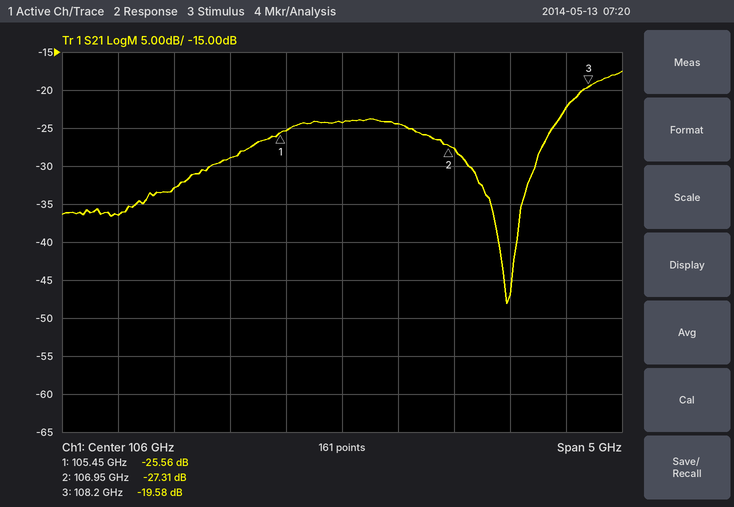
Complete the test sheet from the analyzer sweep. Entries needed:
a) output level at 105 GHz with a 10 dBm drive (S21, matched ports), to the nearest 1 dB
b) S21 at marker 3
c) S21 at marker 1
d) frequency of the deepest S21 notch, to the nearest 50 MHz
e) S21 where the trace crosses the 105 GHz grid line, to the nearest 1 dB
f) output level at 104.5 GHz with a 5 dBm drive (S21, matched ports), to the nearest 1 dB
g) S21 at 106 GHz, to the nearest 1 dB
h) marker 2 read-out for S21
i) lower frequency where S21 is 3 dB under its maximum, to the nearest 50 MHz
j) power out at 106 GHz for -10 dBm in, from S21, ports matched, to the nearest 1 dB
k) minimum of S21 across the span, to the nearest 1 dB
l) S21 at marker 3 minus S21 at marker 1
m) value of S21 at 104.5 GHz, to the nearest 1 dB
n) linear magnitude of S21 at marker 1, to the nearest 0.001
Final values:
-19 dBm
-19.58 dB
-25.56 dB
107.45 GHz
-29 dB
-28 dBm
-24 dB
-27.31 dB
108.10 GHz
-34 dBm
-48 dB
5.98 dB
-33 dB
0.053
